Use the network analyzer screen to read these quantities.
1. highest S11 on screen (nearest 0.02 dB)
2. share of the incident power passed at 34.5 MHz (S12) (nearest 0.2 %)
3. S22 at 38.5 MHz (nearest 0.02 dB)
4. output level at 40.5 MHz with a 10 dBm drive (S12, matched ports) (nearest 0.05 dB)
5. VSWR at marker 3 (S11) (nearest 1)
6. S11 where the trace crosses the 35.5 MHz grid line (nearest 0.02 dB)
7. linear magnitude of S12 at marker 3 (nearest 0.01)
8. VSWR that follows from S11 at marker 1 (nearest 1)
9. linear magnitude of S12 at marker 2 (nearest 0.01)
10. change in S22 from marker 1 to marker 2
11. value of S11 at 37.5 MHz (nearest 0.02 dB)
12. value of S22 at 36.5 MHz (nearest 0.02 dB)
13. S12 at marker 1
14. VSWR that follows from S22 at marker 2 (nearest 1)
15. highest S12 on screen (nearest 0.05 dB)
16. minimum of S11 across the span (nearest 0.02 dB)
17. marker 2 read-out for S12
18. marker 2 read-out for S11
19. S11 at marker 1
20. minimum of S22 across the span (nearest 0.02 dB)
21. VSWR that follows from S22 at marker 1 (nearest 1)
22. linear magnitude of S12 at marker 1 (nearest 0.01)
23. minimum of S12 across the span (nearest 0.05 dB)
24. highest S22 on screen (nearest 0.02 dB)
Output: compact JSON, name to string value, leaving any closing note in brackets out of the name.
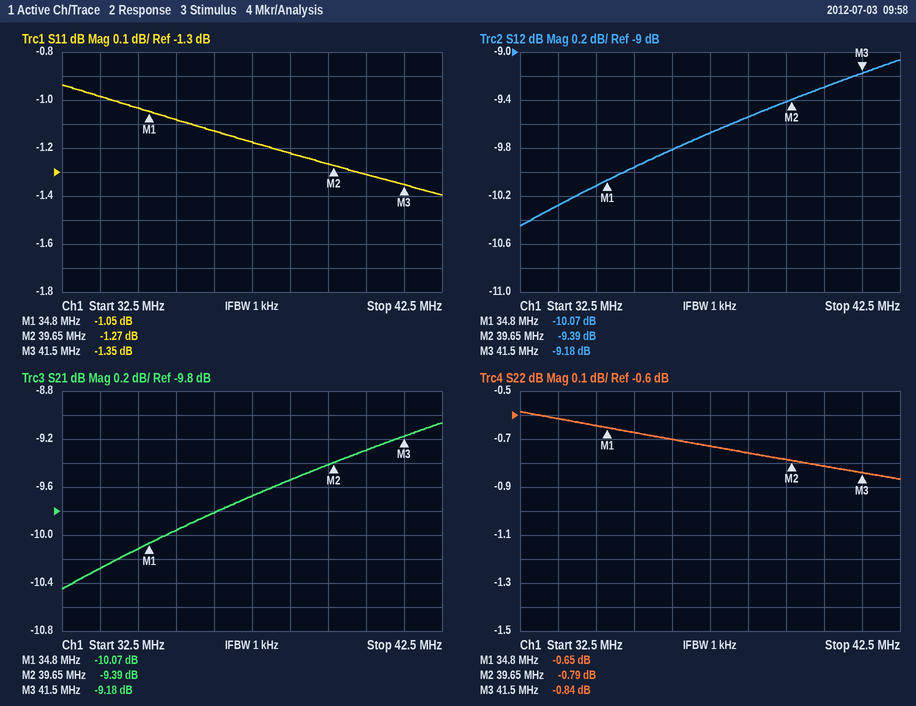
{"highest S11 on screen": "-0.94 dB", "share of the incident power passed at 34.5 MHz (S12)": "9.8 %", "S22 at 38.5 MHz": "-0.76 dB", "output level at 40.5 MHz with a 10 dBm drive (S12, matched ports)": "0.70 dBm", "VSWR at marker 3 (S11)": "13", "S11 where the trace crosses the 35.5 MHz grid line": "-1.08 dB", "linear magnitude of S12 at marker 3": "0.35", "VSWR that follows from S11 at marker 1": "17", "linear magnitude of S12 at marker 2": "0.34", "change in S22 from marker 1 to marker 2": "-0.14 dB", "value of S11 at 37.5 MHz": "-1.18 dB", "value of S22 at 36.5 MHz": "-0.70 dB", "S12 at marker 1": "-10.07 dB", "VSWR that follows from S22 at marker 2": "22", "highest S12 on screen": "-9.05 dB", "minimum of S11 across the span": "-1.40 dB", "marker 2 read-out for S12": "-9.39 dB", "marker 2 read-out for S11": "-1.27 dB", "S11 at marker 1": "-1.05 dB", "minimum of S22 across the span": "-0.86 dB", "VSWR that follows from S22 at marker 1": "27", "linear magnitude of S12 at marker 1": "0.31", "minimum of S12 across the span": "-10.45 dB", "highest S22 on screen": "-0.58 dB"}
